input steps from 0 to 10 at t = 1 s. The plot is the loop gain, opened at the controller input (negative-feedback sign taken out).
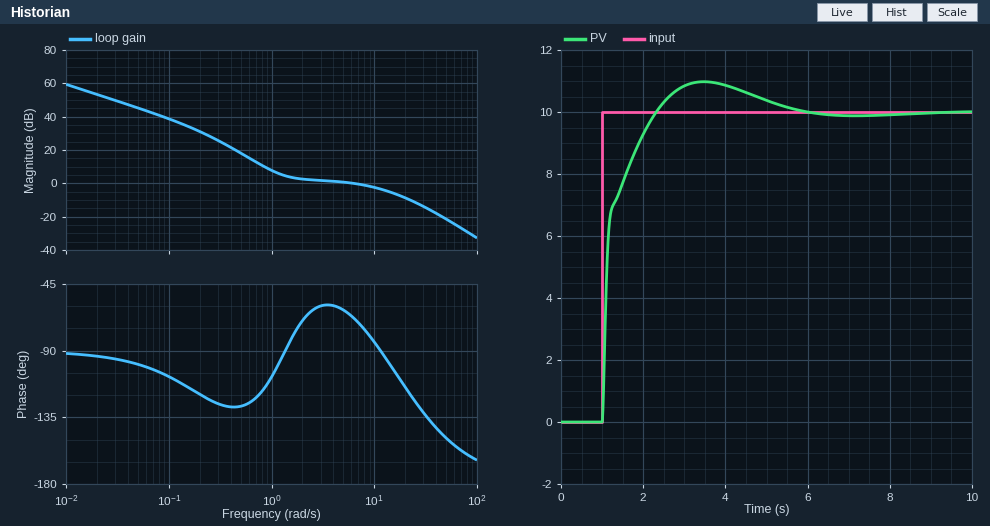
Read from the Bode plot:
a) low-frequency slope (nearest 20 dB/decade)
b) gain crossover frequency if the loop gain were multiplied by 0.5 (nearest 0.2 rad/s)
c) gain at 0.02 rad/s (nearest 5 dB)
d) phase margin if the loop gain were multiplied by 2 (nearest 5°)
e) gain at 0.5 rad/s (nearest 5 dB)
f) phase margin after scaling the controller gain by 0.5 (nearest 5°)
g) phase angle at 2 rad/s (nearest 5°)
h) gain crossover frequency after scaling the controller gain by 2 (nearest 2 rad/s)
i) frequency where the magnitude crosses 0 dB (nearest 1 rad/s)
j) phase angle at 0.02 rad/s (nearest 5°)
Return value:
-20 dB/decade
1.2 rad/s
55 dB
75°
20 dB
80°
-70°
16 rad/s
6 rad/s
-95°
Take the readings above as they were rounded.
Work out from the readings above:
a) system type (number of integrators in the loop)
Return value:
1
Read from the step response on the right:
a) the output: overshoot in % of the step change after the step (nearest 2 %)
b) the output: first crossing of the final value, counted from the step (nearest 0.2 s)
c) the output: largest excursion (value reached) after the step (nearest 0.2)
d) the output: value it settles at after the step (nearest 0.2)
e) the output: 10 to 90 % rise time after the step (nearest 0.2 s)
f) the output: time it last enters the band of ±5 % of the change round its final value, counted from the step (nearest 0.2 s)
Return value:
10 %
1.4 s
11.0
10.0
0.8 s
3.8 s
